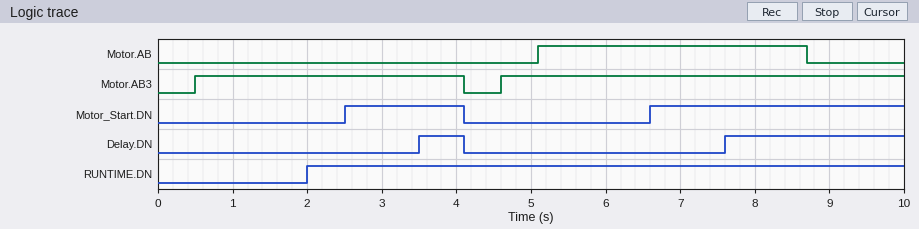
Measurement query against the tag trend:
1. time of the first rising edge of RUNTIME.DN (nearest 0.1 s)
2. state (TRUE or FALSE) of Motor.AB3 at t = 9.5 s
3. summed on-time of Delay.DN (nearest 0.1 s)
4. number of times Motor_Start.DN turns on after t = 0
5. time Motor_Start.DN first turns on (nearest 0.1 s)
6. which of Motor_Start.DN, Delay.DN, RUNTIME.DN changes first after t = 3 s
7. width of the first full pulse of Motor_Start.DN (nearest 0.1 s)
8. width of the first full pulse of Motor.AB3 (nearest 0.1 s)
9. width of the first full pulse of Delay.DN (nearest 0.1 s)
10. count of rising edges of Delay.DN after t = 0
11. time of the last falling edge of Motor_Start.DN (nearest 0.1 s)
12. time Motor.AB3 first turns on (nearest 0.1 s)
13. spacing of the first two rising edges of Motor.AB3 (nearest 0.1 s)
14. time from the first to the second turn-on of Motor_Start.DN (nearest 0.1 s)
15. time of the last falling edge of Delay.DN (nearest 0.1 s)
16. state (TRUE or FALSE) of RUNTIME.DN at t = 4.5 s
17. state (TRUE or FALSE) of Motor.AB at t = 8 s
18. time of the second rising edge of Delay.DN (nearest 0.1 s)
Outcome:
2.0 s
TRUE
3.0 s
2
2.5 s
Delay.DN
1.6 s
3.6 s
0.6 s
2
4.1 s
0.5 s
4.1 s
4.1 s
4.1 s
TRUE
TRUE
7.6 s
